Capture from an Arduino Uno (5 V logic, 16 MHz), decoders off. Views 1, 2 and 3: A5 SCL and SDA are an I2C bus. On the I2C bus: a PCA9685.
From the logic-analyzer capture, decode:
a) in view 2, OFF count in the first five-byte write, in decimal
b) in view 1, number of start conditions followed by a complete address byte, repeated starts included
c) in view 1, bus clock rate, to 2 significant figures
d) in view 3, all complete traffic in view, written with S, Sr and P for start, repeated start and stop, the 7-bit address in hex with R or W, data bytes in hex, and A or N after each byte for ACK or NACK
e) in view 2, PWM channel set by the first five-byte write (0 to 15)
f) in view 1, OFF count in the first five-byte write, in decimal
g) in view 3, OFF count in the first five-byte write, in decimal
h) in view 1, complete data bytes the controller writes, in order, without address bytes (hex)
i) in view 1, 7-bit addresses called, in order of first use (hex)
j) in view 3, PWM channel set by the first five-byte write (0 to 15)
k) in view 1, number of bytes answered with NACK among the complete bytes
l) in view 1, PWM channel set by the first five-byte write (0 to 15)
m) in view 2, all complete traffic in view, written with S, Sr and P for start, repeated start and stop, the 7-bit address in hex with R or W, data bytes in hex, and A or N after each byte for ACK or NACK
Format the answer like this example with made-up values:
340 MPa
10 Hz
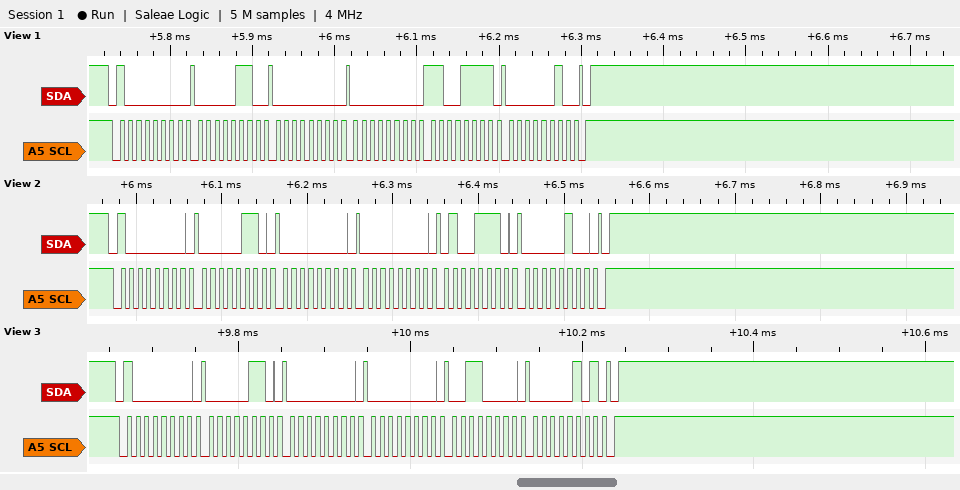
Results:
1102
1
100 kHz
S 40W A 06 A 00 A 00 A 30 A 05 A P
0
719
1328
06 00 00 CF 02
0x40
0
0
0
S 40W A 06 A 00 A 00 A 4E A 04 A P
